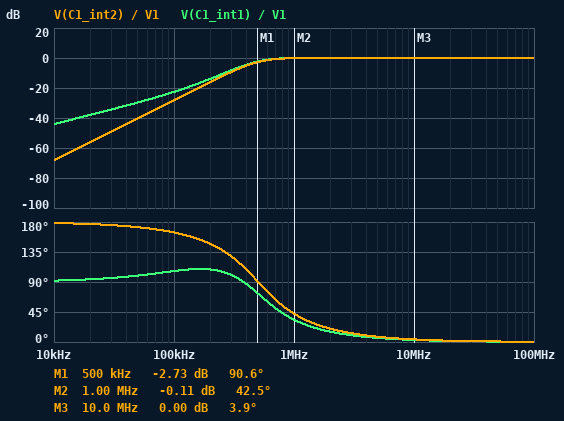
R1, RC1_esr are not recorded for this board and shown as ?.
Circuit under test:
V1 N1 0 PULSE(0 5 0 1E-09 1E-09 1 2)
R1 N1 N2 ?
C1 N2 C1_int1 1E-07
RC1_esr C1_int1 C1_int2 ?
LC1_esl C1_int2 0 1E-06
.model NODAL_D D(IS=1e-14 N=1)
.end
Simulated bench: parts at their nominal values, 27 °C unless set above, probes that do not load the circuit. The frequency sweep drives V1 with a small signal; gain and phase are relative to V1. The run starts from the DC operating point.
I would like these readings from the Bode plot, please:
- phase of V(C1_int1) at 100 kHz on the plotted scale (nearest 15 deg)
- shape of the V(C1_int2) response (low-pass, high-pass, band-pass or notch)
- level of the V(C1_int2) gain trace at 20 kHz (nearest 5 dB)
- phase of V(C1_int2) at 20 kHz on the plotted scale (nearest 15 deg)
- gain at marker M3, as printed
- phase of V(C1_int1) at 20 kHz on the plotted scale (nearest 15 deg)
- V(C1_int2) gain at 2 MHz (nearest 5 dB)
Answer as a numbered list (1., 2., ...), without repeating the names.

1. 105 deg
2. high-pass
3. -55 dB
4. 180 deg
5. 0.00 dB
6. 90 deg
7. 0 dB
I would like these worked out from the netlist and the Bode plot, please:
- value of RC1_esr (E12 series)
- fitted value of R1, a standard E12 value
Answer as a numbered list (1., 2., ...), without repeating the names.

1. 1 Ω
2. 3.3 Ω
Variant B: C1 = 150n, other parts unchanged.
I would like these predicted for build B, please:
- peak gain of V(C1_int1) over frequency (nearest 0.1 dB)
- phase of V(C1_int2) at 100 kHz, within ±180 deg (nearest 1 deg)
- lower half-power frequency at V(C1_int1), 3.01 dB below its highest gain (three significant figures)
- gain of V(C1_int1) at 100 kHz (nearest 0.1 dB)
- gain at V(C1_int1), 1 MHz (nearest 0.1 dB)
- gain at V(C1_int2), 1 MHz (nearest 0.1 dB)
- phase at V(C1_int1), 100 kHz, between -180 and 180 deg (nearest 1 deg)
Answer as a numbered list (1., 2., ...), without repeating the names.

1. 0 dB
2. 157 deg
3. 462 kHz
4. -19.3 dB
5. -0.5 dB
6. -0.6 dB
7. 99 deg
